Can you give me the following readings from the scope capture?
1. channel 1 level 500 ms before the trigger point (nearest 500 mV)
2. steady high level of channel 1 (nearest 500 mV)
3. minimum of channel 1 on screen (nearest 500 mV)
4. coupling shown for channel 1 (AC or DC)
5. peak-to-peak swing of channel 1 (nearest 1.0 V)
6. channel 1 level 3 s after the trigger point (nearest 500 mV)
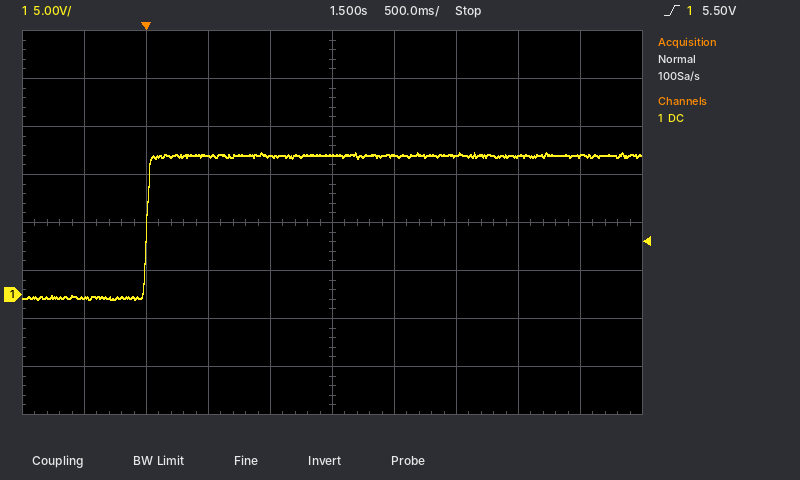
-500 mV
14.5 V
-500 mV
DC
15.0 V
14.5 V
